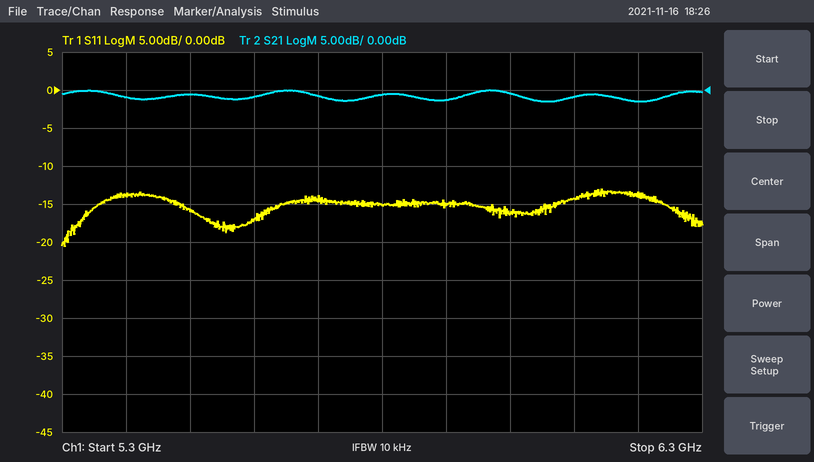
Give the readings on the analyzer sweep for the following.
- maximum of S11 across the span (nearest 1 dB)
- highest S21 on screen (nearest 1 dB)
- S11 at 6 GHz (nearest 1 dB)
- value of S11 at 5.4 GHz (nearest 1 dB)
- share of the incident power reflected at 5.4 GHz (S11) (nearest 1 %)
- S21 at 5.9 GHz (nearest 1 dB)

-13 dB
0 dB
-16 dB
-14 dB
4 %
-1 dB
